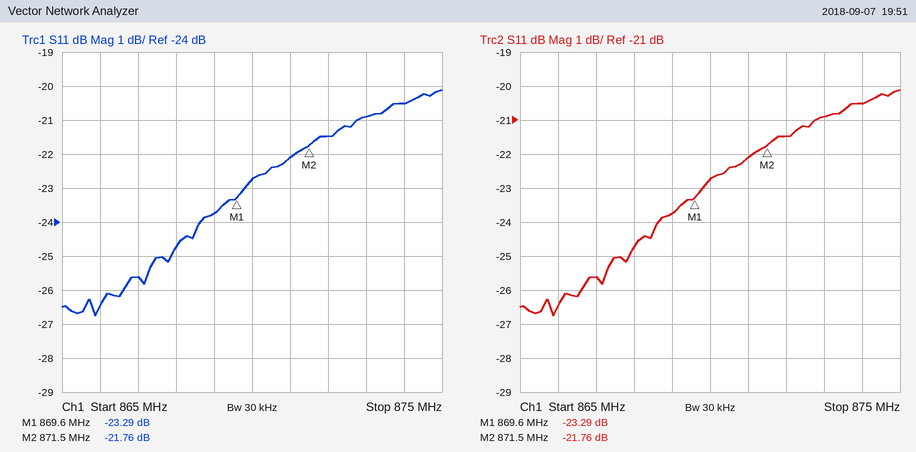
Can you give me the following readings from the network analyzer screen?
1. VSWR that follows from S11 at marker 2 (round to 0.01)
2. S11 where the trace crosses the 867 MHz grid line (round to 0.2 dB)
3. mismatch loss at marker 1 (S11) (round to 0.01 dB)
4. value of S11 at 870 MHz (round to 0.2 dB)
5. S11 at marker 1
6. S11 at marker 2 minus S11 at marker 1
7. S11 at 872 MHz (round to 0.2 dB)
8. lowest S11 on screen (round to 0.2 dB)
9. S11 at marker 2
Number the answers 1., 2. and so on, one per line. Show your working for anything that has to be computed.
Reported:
1. (1 + 0.0817)/(1 − 0.0817) ≈ 1.18
2. -25.6 dB
3. −10 log10(1 − 10^(-23.29/10)) ≈ 0.02 dB
4. -22.8 dB
5. -23.29 dB
6. -21.76 − (-23.29) = 1.53 dB
7. -21.4 dB
8. -26.8 dB
9. -21.76 dB
